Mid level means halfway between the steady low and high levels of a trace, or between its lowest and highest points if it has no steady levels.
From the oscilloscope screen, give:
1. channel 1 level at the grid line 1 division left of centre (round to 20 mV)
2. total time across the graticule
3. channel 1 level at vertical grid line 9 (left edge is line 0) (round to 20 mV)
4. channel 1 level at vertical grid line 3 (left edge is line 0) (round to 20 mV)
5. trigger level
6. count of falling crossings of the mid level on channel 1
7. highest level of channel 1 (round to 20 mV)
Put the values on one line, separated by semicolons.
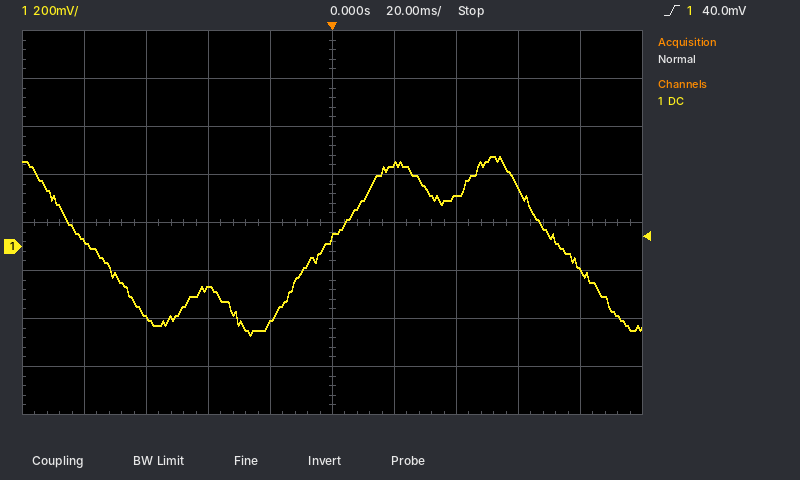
-320 mV; 200 ms; -100 mV; -180 mV; 40.0 mV; 2; 380 mV
